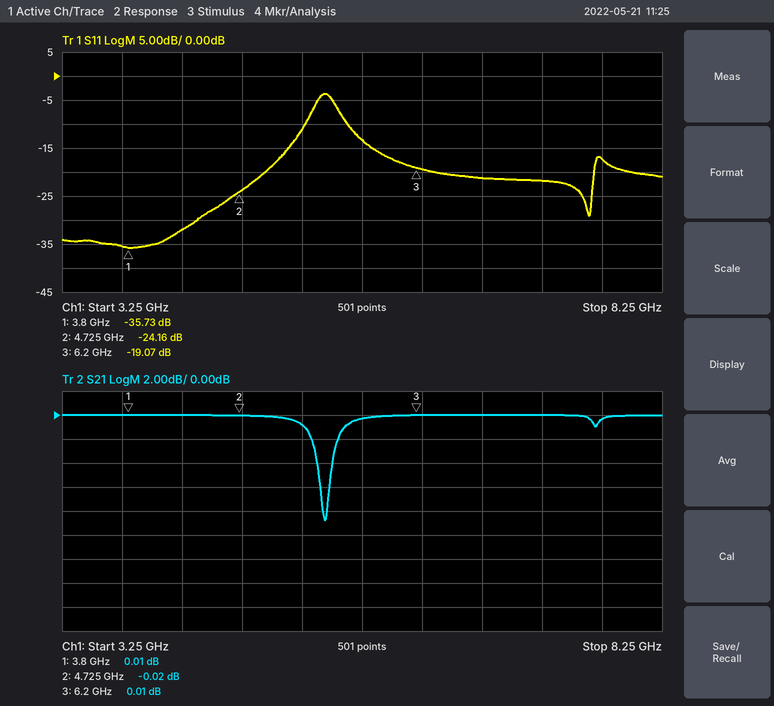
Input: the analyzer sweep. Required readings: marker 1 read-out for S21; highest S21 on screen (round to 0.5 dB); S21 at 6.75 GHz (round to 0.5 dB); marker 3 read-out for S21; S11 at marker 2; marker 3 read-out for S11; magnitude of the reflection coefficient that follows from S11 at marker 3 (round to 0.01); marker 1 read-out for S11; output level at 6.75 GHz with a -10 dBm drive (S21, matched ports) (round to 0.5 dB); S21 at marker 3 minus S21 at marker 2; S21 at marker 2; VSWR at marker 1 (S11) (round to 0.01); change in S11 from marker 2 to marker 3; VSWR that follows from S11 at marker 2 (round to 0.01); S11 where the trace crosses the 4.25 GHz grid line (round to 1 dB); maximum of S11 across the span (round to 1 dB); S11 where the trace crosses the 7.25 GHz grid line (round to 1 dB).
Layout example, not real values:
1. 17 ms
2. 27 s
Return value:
1. 0.01 dB
2. 0.0 dB
3. 0.0 dB
4. 0.01 dB
5. -24.16 dB
6. -19.07 dB
7. 0.11
8. -35.73 dB
9. -10.0 dBm
10. 0.03 dB
11. -0.02 dB
12. 1.03
13. 5.09 dB
14. 1.13
15. -32 dB
16. -4 dB
17. -22 dB
